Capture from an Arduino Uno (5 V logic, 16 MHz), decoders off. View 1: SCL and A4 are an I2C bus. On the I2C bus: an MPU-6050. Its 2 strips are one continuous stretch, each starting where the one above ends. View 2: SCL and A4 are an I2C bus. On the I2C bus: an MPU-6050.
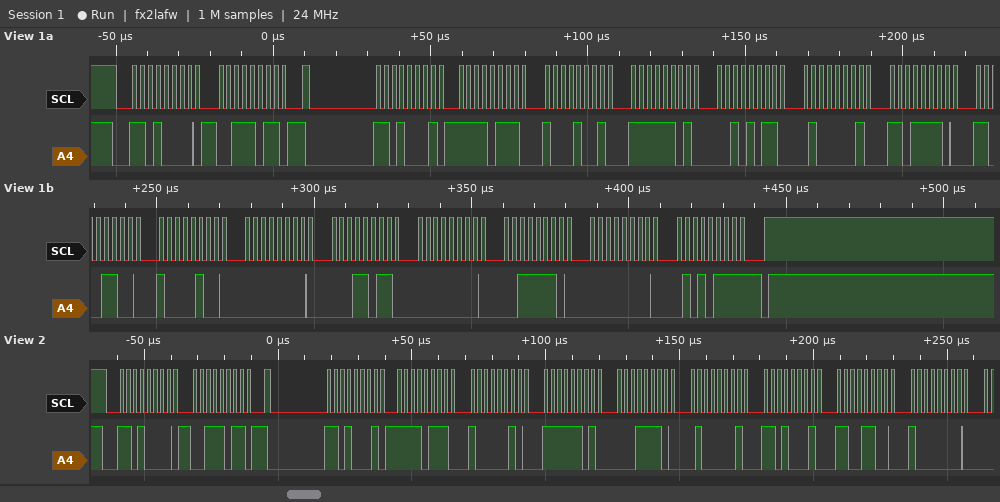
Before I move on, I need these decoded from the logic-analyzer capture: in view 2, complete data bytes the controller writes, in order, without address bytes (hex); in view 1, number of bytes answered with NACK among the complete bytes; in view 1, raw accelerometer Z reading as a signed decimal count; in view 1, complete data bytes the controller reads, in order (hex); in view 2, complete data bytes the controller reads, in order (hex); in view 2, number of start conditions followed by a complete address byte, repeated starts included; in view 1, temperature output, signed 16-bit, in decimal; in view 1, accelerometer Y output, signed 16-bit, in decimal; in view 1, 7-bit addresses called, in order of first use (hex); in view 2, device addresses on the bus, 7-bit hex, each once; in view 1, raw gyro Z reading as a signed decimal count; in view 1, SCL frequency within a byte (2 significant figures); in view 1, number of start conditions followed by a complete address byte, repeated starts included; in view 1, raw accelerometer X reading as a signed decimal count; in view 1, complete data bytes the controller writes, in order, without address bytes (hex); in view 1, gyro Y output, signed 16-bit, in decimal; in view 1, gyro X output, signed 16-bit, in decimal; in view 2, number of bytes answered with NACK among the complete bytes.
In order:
3B
1
16862
F7 89 FD 2B 41 DE CC 84 00 1B 00 3E 00 57
F7 82 FD 1E 41 D1 CC 80
2
-13180
-725
0x68
0x68
87
400 kHz
2
-2167
3B
62
27
0
